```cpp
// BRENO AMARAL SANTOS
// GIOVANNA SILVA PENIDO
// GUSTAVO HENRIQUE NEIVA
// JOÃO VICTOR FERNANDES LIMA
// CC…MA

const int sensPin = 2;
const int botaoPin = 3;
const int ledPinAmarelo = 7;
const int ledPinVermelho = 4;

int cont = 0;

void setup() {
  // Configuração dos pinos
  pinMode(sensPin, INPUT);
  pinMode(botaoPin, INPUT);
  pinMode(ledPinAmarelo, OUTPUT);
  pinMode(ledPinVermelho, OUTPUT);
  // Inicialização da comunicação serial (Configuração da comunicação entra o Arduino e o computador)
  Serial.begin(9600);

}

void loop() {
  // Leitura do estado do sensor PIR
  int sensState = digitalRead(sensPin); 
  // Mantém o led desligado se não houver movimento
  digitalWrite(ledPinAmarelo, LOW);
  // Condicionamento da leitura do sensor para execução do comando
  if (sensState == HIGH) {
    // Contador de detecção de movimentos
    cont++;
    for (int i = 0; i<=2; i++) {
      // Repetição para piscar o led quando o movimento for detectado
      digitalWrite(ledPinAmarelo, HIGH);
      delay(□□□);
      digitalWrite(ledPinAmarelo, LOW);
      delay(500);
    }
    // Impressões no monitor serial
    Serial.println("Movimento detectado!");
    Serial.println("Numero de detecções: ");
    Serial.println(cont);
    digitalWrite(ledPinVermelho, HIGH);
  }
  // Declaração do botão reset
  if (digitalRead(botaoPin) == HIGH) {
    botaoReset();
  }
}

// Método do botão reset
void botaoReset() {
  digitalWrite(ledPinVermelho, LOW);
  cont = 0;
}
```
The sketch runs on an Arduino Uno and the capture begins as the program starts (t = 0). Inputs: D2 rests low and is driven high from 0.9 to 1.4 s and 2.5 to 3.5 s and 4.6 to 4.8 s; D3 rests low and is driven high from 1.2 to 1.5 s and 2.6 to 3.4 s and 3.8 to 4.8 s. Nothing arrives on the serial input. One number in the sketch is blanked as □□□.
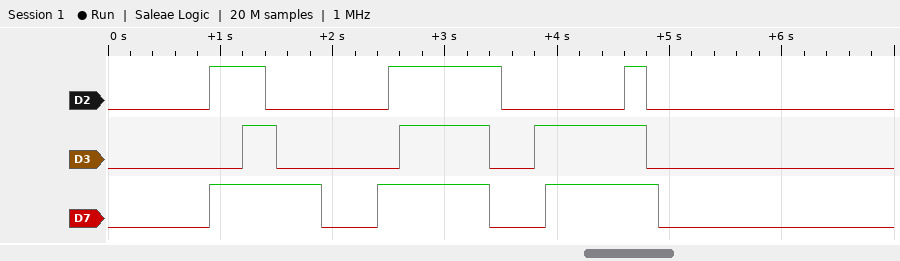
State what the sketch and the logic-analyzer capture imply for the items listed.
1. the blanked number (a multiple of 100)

1000
